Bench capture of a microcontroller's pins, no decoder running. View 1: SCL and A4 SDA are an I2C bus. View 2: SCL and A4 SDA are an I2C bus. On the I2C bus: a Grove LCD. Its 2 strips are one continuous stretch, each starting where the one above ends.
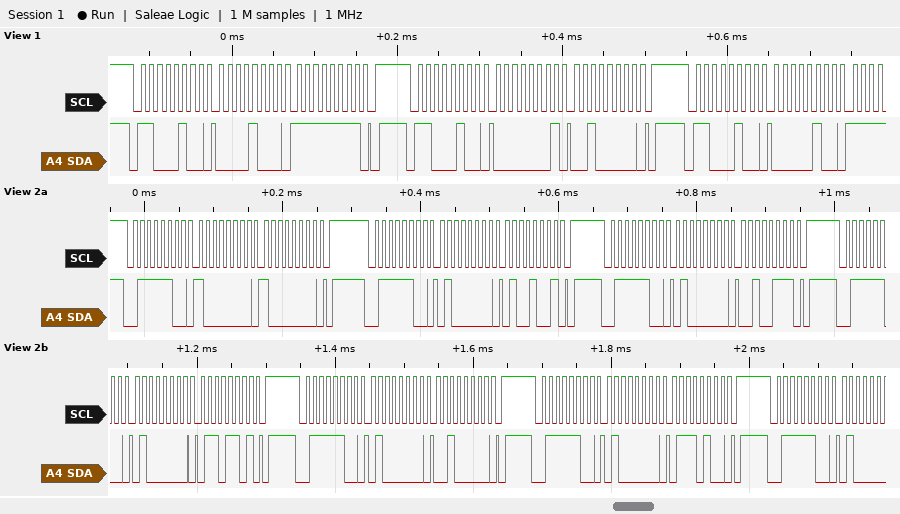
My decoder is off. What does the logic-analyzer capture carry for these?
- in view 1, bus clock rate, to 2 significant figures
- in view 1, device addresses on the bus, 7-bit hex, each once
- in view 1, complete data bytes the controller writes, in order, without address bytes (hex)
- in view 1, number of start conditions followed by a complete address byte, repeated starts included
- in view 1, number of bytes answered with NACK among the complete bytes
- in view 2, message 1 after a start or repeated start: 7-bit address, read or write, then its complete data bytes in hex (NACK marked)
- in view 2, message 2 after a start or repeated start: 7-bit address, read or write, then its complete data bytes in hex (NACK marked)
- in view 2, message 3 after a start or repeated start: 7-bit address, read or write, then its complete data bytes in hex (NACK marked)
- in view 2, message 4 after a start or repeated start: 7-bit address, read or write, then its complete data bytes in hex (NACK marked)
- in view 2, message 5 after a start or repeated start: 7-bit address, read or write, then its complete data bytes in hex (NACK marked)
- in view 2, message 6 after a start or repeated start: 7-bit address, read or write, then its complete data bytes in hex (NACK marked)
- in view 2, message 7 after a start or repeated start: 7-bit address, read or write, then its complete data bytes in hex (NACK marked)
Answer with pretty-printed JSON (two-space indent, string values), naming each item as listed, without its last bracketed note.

{
  "in view 1, bus clock rate, to 2 significant figures": "100 kHz",
  "in view 1, device addresses on the bus, 7-bit hex, each once": "0x62",
  "in view 1, complete data bytes the controller writes, in order, without address bytes": "08 FF 01 20 04",
  "in view 1, number of start conditions followed by a complete address byte, repeated starts included": "3",
  "in view 1, number of bytes answered with NACK among the complete bytes": "0",
  "in view 2, message 1 after a start or repeated start: 7-bit address, read or write, then its complete data bytes in hex": "0x3E write: 80 80",
  "in view 2, message 2 after a start or repeated start: 7-bit address, read or write, then its complete data bytes in hex": "0x3E write: 40 49",
  "in view 2, message 3 after a start or repeated start: 7-bit address, read or write, then its complete data bytes in hex": "0x3E write: 40 27",
  "in view 2, message 4 after a start or repeated start: 7-bit address, read or write, then its complete data bytes in hex": "0x3E write: 40 6D",
  "in view 2, message 5 after a start or repeated start: 7-bit address, read or write, then its complete data bytes in hex": "0x3E write: 40 20",
  "in view 2, message 6 after a start or repeated start: 7-bit address, read or write, then its complete data bytes in hex": "0x3E write: 40 74",
  "in view 2, message 7 after a start or repeated start: 7-bit address, read or write, then its complete data bytes in hex": "0x3E write"
}
